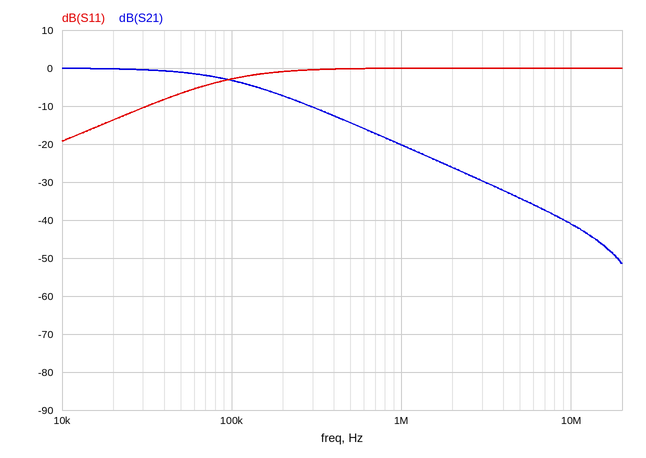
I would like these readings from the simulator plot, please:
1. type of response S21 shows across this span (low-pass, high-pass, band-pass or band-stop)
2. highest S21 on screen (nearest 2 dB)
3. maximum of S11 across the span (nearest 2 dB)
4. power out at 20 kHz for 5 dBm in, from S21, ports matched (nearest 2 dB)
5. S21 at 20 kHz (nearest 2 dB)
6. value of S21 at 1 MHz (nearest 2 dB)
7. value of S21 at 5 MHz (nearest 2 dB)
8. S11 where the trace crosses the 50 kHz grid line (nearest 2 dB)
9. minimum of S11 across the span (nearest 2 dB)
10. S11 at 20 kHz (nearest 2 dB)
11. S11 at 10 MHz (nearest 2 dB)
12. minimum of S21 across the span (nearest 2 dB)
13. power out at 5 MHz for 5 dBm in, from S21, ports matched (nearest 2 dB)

low-pass
0 dB
0 dB
4 dBm
0 dB
-20 dB
-34 dB
-6 dB
-20 dB
-14 dB
0 dB
-52 dB
-30 dBm
